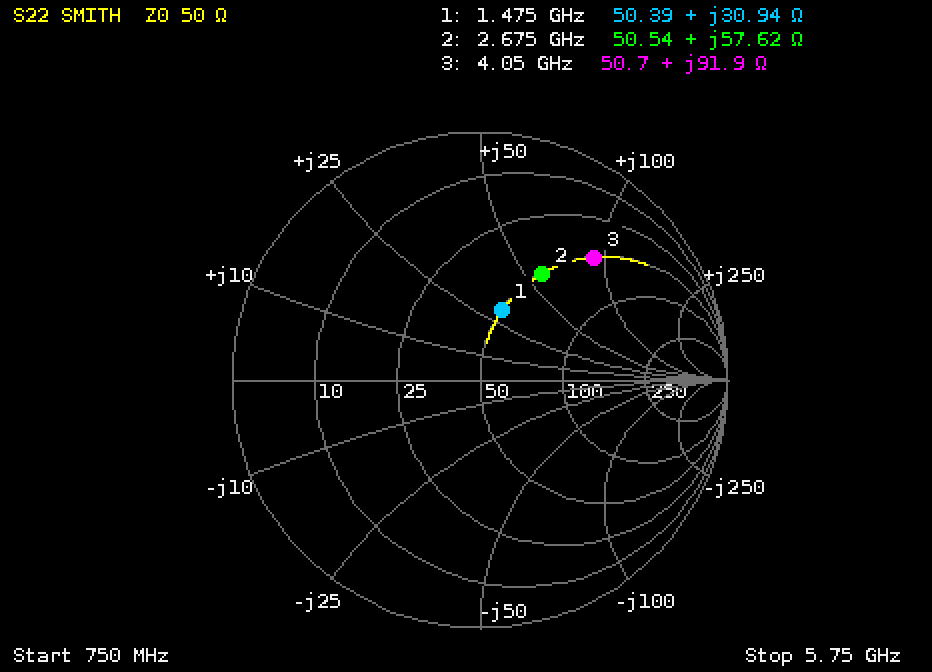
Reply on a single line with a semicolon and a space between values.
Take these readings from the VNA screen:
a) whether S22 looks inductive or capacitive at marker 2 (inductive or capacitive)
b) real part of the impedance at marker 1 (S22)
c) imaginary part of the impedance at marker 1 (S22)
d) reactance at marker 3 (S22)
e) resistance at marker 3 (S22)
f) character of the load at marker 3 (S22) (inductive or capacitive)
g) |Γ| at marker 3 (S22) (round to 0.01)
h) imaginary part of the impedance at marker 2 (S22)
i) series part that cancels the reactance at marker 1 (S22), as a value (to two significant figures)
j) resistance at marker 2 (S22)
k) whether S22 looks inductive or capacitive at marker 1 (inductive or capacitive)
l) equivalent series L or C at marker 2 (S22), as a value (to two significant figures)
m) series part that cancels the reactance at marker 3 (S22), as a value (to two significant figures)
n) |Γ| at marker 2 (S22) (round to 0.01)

inductive; 50.39 Ω; +30.94 Ω; +91.9 Ω; 50.7 Ω; inductive; 0.67; +57.62 Ω; 3.5 pF; 50.54 Ω; inductive; 3.4 nH; 430 fF; 0.50
